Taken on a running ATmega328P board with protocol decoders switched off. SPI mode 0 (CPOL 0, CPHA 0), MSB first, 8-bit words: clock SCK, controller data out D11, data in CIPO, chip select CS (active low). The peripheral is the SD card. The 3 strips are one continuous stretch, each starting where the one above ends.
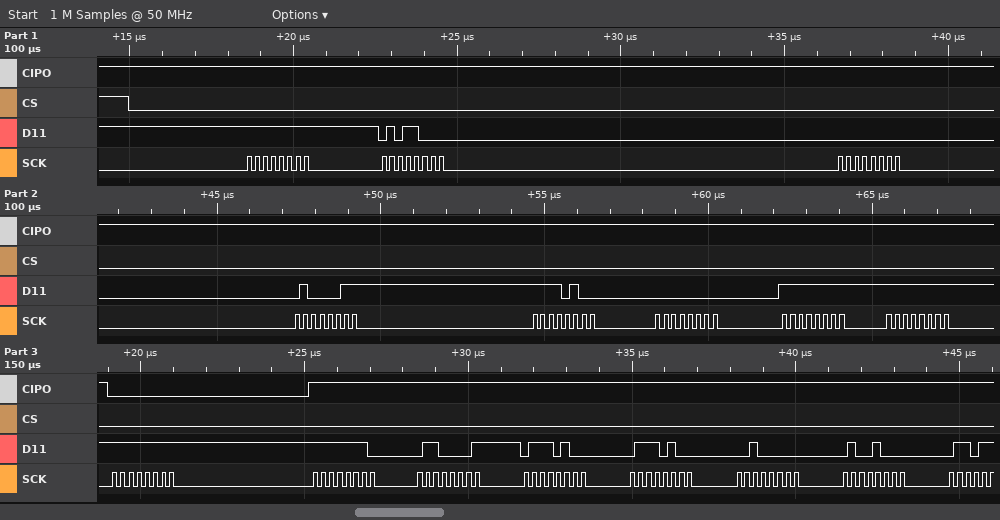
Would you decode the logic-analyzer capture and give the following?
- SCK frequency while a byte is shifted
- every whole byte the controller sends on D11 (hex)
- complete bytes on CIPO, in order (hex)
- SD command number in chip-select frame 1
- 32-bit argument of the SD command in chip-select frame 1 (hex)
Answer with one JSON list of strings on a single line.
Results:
["4 MHz", "FF 58 00 43 F4 00 FF FF FF FE 61 74 74 20 48", "FF FF FF FF FF FF FF FF 00 FF FF FF FF FF FF", "CMD24", "0x0043F400"]
